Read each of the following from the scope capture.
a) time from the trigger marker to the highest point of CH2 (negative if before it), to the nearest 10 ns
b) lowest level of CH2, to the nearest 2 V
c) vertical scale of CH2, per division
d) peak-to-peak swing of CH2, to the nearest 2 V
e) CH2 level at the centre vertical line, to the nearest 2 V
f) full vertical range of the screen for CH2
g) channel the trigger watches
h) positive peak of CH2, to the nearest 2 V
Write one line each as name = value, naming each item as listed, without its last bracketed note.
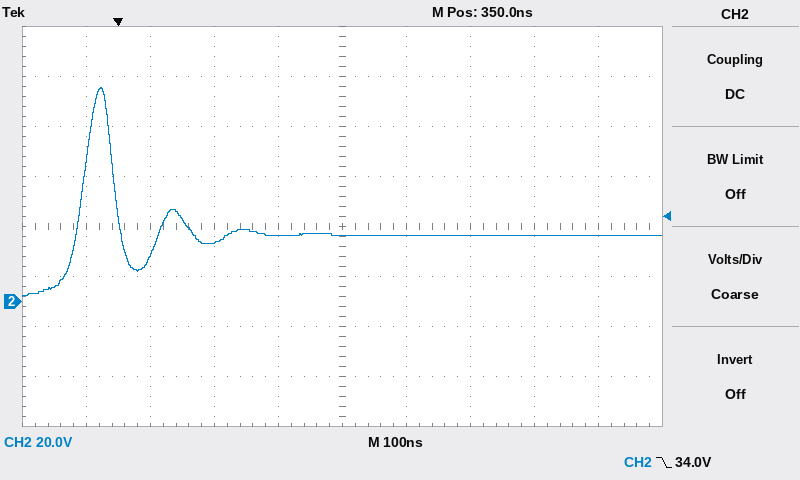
time from the trigger marker to the highest point of CH2 (negative if before it), to the nearest 10 ns = -30 ns
lowest level of CH2, to the nearest 2 V = 2 V
vertical scale of CH2, per division = 20 V
peak-to-peak swing of CH2, to the nearest 2 V = 84 V
CH2 level at the centre vertical line, to the nearest 2 V = 26 V
full vertical range of the screen for CH2 = 160 V
channel the trigger watches = CH2
positive peak of CH2, to the nearest 2 V = 86 V
